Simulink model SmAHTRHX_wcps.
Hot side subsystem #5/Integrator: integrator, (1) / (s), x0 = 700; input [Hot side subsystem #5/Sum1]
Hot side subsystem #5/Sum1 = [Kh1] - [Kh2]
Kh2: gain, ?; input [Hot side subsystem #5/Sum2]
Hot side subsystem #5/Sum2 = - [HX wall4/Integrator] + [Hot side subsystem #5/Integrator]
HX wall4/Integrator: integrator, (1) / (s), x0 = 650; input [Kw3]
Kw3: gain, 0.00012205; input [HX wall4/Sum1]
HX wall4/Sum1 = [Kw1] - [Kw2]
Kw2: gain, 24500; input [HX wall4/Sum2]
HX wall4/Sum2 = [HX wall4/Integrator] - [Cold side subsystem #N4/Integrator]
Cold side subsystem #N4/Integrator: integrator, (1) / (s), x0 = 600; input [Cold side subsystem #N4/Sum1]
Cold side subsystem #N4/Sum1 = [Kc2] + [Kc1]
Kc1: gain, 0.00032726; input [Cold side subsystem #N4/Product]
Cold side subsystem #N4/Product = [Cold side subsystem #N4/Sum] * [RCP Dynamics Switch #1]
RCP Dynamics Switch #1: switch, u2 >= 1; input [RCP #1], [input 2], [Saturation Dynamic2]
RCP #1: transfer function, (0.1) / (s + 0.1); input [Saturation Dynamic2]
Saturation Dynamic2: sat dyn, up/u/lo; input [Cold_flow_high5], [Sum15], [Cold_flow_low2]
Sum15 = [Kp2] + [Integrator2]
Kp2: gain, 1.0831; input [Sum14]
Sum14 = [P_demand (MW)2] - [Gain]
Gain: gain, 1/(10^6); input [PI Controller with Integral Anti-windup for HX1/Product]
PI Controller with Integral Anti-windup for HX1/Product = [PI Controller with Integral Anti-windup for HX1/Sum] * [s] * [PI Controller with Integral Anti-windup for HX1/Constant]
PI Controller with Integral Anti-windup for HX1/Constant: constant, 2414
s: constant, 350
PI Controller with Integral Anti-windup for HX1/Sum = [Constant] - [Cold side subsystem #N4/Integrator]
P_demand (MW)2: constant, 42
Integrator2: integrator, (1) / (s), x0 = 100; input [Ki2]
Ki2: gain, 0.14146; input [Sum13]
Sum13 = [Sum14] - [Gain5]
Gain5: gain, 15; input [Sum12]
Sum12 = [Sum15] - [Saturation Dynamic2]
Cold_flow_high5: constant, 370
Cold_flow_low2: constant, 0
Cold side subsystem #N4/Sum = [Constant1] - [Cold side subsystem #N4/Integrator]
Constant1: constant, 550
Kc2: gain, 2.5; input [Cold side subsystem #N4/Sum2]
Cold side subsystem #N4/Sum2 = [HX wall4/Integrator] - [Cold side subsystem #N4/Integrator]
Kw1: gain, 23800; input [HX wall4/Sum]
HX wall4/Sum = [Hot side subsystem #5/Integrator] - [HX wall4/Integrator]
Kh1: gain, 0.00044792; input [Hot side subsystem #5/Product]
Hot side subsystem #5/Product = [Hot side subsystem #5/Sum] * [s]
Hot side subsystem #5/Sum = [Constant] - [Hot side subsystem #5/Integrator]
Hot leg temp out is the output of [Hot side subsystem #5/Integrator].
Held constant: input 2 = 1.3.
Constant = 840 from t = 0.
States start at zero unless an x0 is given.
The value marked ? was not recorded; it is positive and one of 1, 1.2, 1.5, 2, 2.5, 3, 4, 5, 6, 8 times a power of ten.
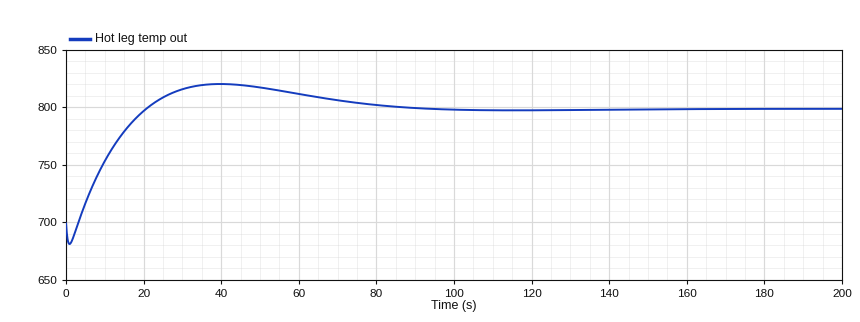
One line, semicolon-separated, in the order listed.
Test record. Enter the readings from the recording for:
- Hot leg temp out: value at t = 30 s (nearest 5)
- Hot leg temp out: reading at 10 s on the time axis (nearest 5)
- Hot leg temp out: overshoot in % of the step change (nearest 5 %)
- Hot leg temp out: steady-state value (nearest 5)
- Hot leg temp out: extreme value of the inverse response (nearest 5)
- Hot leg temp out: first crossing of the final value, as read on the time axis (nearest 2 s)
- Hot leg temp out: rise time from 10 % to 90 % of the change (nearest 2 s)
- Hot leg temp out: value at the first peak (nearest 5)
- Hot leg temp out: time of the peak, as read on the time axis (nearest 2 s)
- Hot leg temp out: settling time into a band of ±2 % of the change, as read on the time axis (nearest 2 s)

815; 755; 20 %; 800; 680; 20 s; 14 s; 820; 40 s; 84 s
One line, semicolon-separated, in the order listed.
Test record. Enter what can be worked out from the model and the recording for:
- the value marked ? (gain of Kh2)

1.5
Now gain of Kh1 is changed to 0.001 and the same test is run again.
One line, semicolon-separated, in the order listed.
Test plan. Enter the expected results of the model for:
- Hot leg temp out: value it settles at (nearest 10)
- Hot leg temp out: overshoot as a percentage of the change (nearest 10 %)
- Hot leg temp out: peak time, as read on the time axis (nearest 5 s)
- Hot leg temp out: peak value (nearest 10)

810; 20 %; 25 s; 830
